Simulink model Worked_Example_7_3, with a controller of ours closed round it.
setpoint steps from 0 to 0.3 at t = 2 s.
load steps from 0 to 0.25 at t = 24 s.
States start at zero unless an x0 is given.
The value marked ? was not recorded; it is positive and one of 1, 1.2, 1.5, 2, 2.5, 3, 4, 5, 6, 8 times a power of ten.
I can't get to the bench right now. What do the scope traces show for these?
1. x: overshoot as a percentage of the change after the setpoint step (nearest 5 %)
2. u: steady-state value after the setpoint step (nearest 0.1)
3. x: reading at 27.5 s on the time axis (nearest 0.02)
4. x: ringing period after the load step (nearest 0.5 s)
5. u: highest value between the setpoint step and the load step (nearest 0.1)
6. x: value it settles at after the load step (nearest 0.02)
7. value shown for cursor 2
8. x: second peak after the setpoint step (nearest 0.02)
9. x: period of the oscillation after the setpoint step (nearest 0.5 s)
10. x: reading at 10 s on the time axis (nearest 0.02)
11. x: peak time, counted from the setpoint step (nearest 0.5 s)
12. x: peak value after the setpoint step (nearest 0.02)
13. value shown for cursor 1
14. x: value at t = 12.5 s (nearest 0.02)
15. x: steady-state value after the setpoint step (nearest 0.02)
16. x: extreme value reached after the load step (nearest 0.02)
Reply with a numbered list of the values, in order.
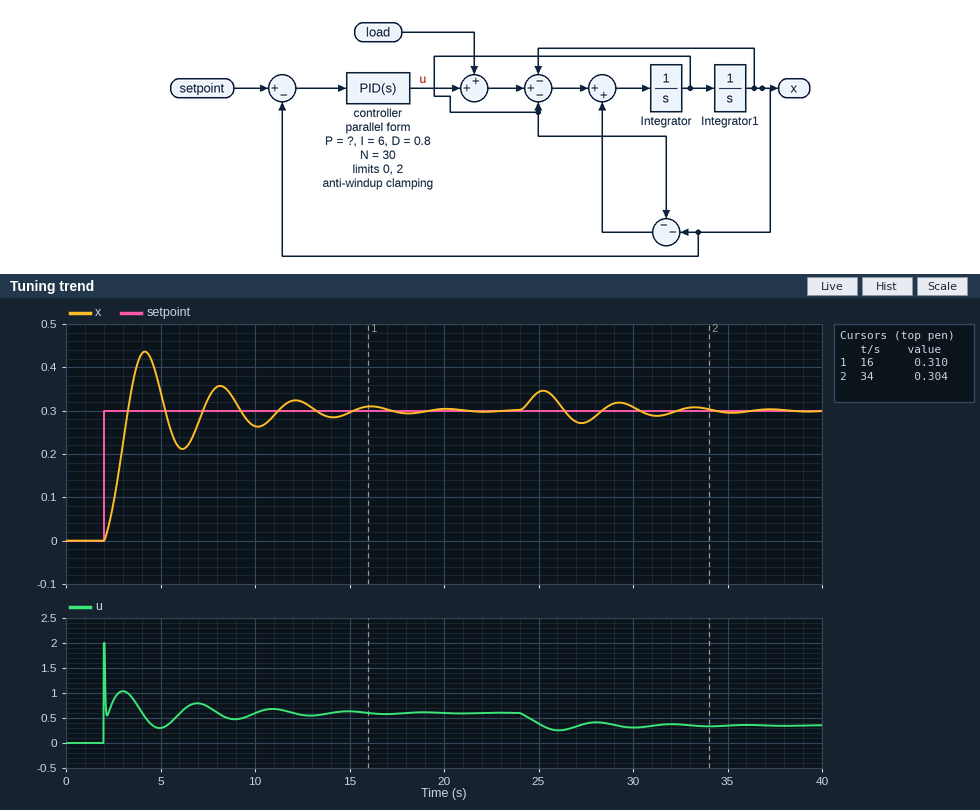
1. 45 %
2. 0.6
3. 0.28
4. 4.0 s
5. 2.0
6. 0.30
7. 0.304
8. 0.36
9. 4.0 s
10. 0.26
11. 2.0 s
12. 0.44
13. 0.310
14. 0.32
15. 0.30
16. 0.34
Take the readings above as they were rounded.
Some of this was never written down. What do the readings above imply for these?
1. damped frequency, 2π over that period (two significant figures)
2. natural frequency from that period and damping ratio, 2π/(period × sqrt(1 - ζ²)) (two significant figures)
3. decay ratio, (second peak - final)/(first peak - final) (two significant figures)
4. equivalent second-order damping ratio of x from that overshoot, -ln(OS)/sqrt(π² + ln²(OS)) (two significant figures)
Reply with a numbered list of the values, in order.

1. 1.6 rad/s
2. 1.6 rad/s
3. 0.43
4. 0.25
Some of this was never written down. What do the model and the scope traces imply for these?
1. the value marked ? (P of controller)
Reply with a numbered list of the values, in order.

1. 1.5
